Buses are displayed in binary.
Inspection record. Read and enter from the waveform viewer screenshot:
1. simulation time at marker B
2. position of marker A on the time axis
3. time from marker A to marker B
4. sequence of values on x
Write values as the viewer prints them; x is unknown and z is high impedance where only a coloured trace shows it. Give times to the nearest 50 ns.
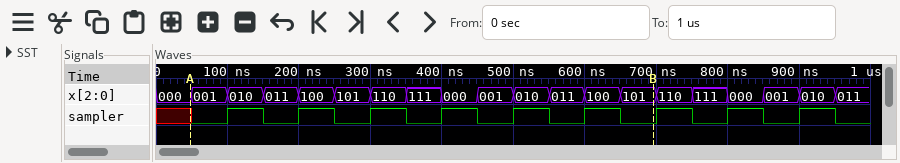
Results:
700 ns
50 ns
650 ns
000, 001, 010, 011, 100, 101, 110, 111, 000, 001, 010, 011, 100, 101, 110, 111, 000, 001, 010, 011
